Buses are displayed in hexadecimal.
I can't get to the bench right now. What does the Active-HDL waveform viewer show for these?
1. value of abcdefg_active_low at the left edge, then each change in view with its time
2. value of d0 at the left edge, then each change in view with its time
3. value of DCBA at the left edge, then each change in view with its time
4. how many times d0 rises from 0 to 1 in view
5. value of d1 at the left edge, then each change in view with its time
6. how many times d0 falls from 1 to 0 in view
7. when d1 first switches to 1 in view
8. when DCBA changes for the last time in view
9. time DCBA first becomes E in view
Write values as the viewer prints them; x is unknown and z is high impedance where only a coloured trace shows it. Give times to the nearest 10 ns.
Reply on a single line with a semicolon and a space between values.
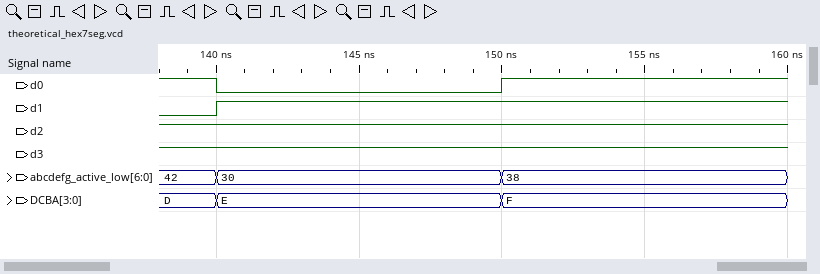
42, 30 at 140 ns, 38 at 150 ns; 1, 0 at 140 ns, 1 at 150 ns; D, E at 140 ns, F at 150 ns; 1; 0, 1 at 140 ns; 1; 140 ns; 150 ns; 140 ns
